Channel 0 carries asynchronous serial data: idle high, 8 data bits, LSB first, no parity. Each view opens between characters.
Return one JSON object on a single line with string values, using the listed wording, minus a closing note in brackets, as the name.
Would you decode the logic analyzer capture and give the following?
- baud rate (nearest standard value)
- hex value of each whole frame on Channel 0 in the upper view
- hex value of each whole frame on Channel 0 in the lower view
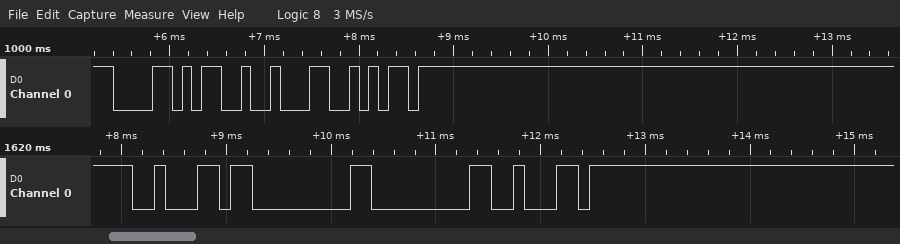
{"baud rate": "9600 baud", "hex value of each whole frame on Channel 0 in the upper view": "58, 12, 6A", "hex value of each whole frame on Channel 0 in the lower view": "62, 00, 00, 62"}
